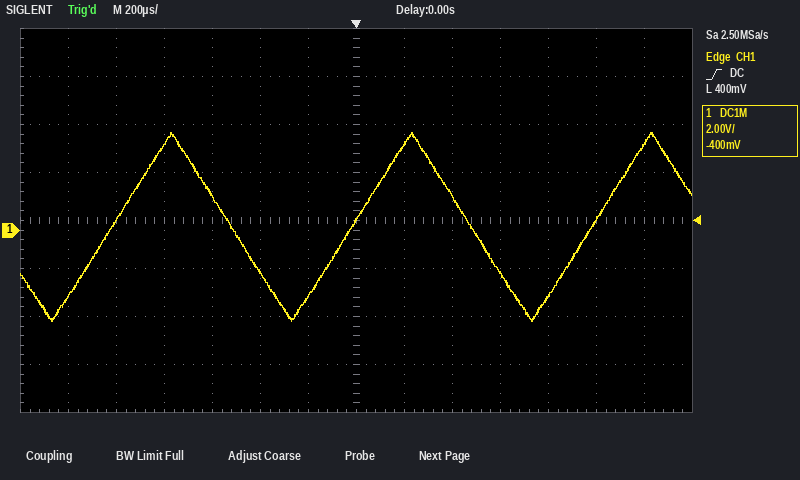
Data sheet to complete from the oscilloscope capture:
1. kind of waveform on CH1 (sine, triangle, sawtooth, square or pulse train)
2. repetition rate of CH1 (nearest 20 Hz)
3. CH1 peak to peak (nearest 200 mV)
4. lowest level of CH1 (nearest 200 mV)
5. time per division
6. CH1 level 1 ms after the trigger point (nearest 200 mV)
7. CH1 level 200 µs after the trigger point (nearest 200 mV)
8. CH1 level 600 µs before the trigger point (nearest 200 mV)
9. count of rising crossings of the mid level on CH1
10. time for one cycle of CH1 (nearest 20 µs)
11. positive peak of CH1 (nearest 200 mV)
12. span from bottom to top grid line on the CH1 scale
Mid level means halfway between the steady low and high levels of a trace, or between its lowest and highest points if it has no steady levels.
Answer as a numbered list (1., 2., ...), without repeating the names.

1. triangle
2. 1.00 kHz
3. 7.8 V
4. -3.8 V
5. 200 µs
6. 400 mV
7. 3.6 V
8. 1.4 V
9. 3
10. 1.00 ms
11. 4.0 V
12. 16 V
